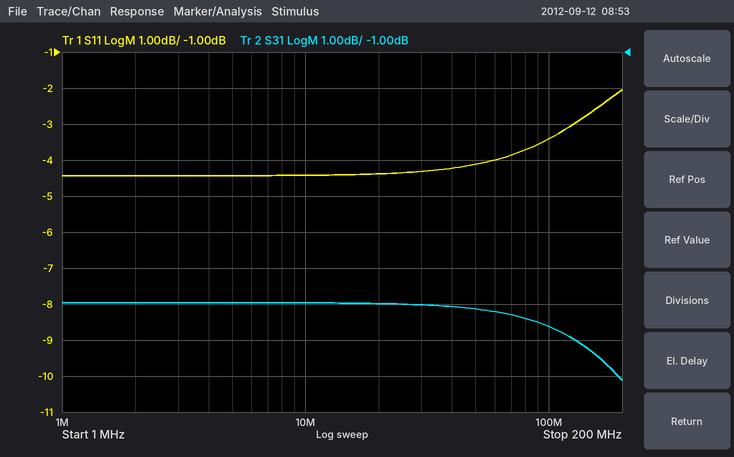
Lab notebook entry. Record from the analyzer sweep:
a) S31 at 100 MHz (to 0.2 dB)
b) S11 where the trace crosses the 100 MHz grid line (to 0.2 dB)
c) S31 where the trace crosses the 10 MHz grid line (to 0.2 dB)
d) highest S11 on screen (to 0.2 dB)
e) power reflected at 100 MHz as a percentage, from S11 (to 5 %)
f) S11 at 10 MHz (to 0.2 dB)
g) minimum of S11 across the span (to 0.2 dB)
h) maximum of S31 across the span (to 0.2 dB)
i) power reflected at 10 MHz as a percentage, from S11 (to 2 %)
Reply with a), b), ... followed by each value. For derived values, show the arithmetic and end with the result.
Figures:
a) -8.6 dB
b) -3.4 dB
c) -8.0 dB
d) -2.0 dB
e) 10^(-3.4/10) ≈ 45.7 %, so 45 % to the nearest 5 %
f) -4.4 dB
g) -4.4 dB
h) -8.0 dB
i) 10^(-4.4/10) ≈ 36 %
